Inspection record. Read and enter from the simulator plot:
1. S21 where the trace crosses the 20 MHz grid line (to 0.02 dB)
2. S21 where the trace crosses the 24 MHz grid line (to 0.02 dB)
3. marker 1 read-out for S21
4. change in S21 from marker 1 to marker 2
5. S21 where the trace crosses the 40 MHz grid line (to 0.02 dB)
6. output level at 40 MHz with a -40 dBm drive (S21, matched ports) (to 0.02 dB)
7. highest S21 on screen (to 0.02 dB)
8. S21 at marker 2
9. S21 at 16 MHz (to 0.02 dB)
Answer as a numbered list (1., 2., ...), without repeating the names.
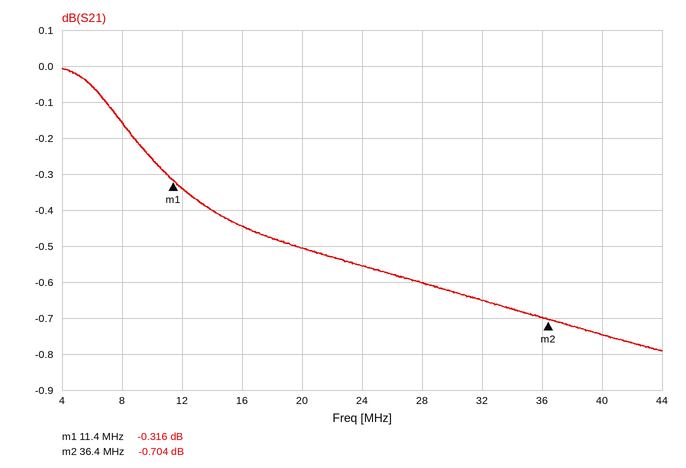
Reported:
1. -0.50 dB
2. -0.56 dB
3. -0.316 dB
4. -0.388 dB
5. -0.74 dB
6. -40.74 dBm
7. 0.00 dB
8. -0.704 dB
9. -0.44 dB
